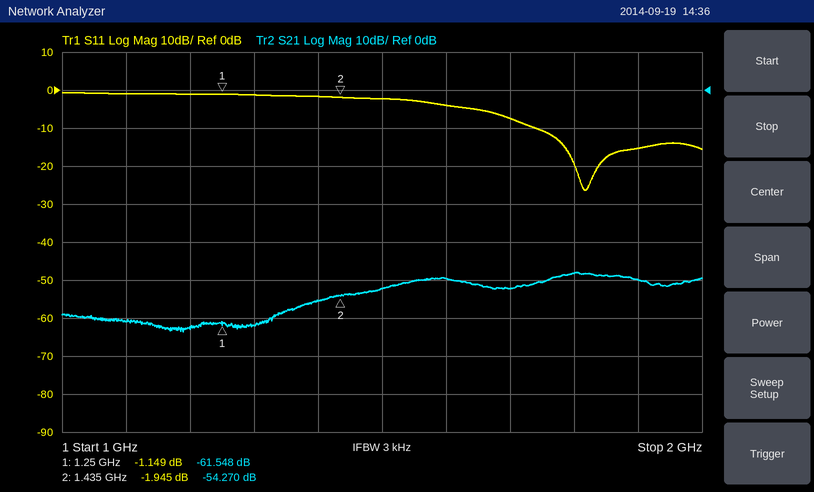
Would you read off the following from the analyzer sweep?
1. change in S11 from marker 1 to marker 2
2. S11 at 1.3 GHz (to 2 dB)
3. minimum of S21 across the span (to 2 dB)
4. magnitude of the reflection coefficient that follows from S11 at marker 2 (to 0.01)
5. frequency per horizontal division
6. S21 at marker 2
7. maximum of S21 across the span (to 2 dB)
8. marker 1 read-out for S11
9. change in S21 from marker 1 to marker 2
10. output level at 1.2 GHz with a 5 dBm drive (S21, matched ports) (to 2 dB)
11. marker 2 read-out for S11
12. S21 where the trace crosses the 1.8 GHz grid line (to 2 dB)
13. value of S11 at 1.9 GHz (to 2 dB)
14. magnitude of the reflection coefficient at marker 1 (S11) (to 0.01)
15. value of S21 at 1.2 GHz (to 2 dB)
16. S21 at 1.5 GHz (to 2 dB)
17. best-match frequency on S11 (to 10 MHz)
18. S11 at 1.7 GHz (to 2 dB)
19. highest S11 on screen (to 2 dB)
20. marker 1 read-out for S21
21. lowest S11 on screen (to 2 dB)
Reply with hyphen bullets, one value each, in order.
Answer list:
- -0.796 dB
- -2 dB
- -64 dB
- 0.80
- 100 MHz
- -54.270 dB
- -48 dB
- -1.149 dB
- 7.278 dB
- -58 dBm
- -1.945 dB
- -48 dB
- -16 dB
- 0.88
- -62 dB
- -52 dB
- 1.82 GHz
- -8 dB
- 0 dB
- -61.548 dB
- -26 dB
